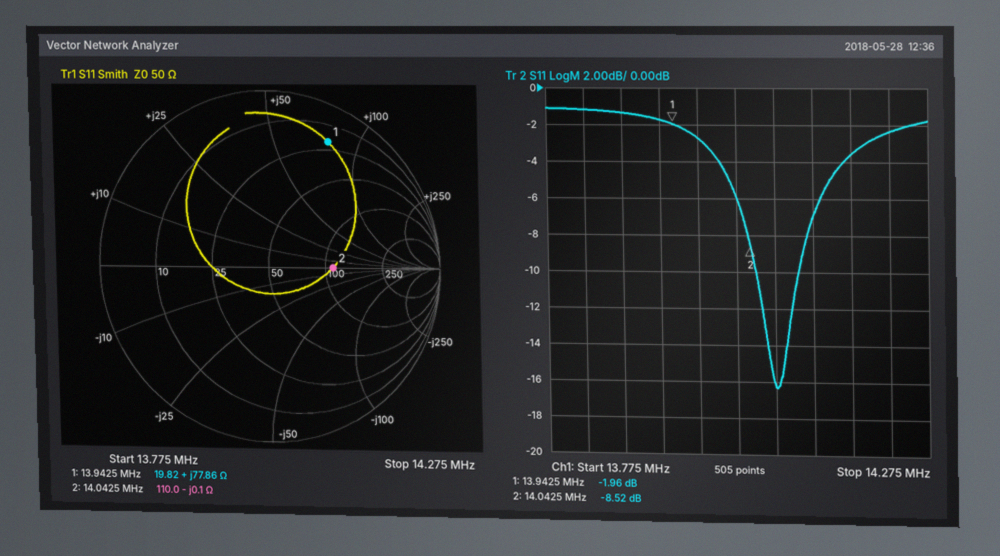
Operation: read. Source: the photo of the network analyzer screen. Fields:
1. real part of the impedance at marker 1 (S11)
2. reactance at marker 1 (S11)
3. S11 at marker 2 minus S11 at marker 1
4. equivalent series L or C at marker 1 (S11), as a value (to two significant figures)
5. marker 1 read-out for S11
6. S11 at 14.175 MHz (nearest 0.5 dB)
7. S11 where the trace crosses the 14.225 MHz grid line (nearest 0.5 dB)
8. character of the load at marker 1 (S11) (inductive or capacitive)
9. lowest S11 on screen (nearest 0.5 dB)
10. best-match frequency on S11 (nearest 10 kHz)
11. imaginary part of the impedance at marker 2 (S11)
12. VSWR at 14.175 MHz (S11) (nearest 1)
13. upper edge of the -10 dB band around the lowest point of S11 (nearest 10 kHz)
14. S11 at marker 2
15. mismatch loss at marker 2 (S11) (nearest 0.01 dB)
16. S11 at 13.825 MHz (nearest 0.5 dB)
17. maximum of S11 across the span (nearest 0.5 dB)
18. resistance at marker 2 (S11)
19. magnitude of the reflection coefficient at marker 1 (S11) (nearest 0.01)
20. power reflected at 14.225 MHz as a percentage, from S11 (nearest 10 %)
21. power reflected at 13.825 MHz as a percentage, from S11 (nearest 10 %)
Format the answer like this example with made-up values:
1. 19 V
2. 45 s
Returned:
1. 19.82 Ω
2. +77.86 Ω
3. -6.56 dB
4. 890 nH
5. -1.96 dB
6. -3.5 dB
7. -2.5 dB
8. inductive
9. -16.5 dB
10. 14.08 MHz
11. -0.1 Ω
12. 5
13. 14.11 MHz
14. -8.52 dB
15. 0.66 dB
16. -1.0 dB
17. -1.0 dB
18. 110.0 Ω
19. 0.80
20. 60 %
21. 80 %
